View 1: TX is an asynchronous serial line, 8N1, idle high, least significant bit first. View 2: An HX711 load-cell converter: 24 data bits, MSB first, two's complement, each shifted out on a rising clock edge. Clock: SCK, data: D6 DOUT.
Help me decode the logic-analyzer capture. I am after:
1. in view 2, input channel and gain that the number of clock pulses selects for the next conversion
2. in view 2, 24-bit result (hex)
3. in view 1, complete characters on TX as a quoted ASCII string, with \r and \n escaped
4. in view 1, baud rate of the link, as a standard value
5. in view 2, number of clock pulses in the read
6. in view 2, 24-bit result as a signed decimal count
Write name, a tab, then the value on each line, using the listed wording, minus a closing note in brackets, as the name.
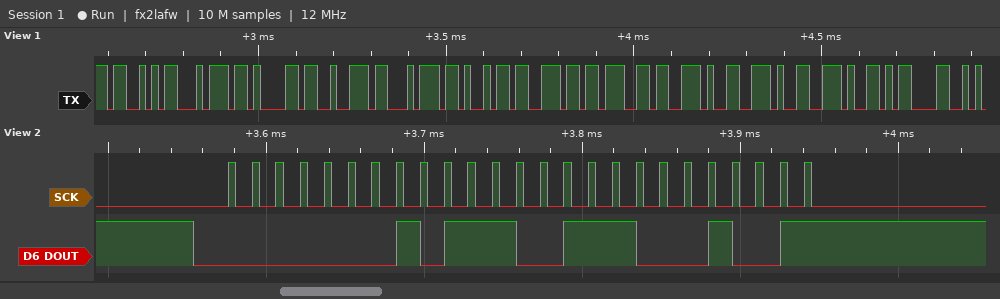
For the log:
in view 2, input channel and gain that the number of clock pulses selects for the next conversion	channel A, gain 128
in view 2, 24-bit result	0x017389
in view 1, complete characters on TX as a quoted ASCII string, with \r and \n escaped	"Starting...\r"
in view 1, baud rate of the link, as a standard value	57600 baud
in view 2, number of clock pulses in the read	25
in view 2, 24-bit result as a signed decimal count	95113
